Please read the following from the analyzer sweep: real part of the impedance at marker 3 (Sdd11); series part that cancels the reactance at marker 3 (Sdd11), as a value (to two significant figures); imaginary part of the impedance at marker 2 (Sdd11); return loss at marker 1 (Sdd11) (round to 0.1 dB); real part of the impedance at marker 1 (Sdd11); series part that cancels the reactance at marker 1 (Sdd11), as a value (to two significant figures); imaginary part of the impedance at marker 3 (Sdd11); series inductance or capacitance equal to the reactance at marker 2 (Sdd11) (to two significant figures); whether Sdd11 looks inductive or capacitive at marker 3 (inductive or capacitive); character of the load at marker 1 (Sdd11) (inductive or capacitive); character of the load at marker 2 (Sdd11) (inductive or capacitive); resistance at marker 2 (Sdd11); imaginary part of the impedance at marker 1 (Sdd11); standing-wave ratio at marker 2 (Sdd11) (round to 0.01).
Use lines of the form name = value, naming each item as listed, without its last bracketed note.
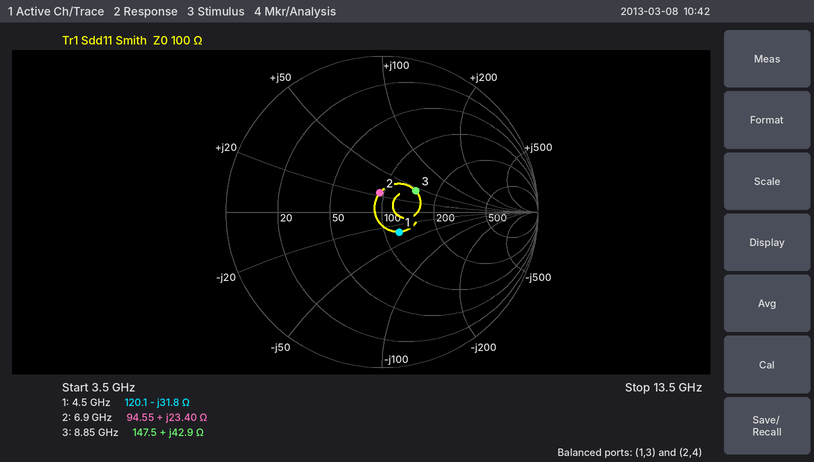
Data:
real part of the impedance at marker 3 = 147.5 Ω
series part that cancels the reactance at marker 3 (Sdd11), as a value = 420 fF
imaginary part of the impedance at marker 2 = +23.40 Ω
return loss at marker 1 (Sdd11) = 15.4 dB
real part of the impedance at marker 1 = 120.1 Ω
series part that cancels the reactance at marker 1 (Sdd11), as a value = 1.1 nH
imaginary part of the impedance at marker 3 = +42.9 Ω
series inductance or capacitance equal to the reactance at marker 2 (Sdd11) = 540 pH
whether Sdd11 looks inductive or capacitive at marker 3 = inductive
character of the load at marker 1 (Sdd11) = capacitive
character of the load at marker 2 (Sdd11) = inductive
resistance at marker 2 = 94.55 Ω
imaginary part of the impedance at marker 1 = -31.8 Ω
standing-wave ratio at marker 2 (Sdd11) = 1.28
